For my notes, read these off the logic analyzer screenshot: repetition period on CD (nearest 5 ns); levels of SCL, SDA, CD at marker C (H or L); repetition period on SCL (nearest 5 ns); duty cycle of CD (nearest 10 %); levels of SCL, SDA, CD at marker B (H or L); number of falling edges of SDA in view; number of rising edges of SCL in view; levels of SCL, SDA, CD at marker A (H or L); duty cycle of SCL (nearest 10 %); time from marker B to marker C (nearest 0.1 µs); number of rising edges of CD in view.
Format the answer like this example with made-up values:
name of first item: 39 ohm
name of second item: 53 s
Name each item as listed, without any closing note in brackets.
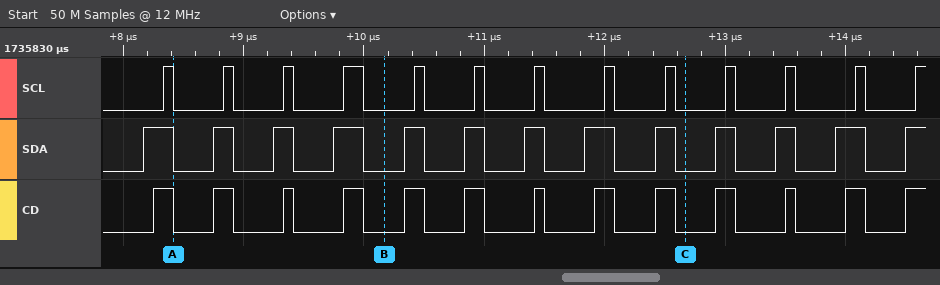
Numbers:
repetition period on CD: 520 ns
levels of SCL, SDA, CD at marker C: SCL=L, SDA=L, CD=L
repetition period on SCL: 520 ns
duty cycle of CD: 30 %
levels of SCL, SDA, CD at marker B: SCL=L, SDA=L, CD=L
number of falling edges of SDA in view: 12
number of rising edges of SCL in view: 13
levels of SCL, SDA, CD at marker A: SCL=L, SDA=L, CD=L
duty cycle of SCL: 20 %
time from marker B to marker C: 2.5 µs
number of rising edges of CD in view: 13
